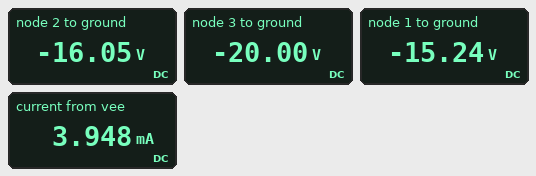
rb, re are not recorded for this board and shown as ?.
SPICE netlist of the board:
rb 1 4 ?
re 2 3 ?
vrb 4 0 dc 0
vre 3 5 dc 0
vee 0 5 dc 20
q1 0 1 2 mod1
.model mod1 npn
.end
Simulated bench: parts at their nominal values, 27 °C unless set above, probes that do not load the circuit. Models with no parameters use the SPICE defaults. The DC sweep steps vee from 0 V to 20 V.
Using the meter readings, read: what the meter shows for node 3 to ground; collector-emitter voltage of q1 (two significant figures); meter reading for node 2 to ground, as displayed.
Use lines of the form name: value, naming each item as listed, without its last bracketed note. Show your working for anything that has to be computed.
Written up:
what the meter shows for node 3 to ground: -20.00 V
collector-emitter voltage of q1: 0 V - (-16.05 V) = 16 V
meter reading for node 2 to ground, as displayed: -16.05 V
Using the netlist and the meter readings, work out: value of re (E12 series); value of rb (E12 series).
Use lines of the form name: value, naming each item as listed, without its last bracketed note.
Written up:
value of re: 1 kΩ
value of rb: 390 kΩ
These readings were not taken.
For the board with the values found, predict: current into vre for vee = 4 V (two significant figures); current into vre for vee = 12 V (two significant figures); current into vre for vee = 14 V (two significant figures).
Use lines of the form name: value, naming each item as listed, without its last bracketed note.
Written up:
current into vre for vee = 4 V: 670 µA
current into vre for vee = 12 V: 2.3 mA
current into vre for vee = 14 V: 2.7 mA
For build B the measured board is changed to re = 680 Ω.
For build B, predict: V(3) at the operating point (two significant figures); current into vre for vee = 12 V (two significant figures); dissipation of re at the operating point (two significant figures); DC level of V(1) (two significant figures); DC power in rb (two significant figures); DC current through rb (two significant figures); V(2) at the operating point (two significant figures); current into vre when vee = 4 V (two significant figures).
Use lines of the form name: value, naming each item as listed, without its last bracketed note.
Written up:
V(3) at the operating point: -20 V
current into vre for vee = 12 V: 2.5 mA
dissipation of re at the operating point: 12 mW
DC level of V(1): -16 V
DC power in rb: 680 µW
DC current through rb: 42 µA
V(2) at the operating point: -17 V
current into vre when vee = 4 V: 710 µA
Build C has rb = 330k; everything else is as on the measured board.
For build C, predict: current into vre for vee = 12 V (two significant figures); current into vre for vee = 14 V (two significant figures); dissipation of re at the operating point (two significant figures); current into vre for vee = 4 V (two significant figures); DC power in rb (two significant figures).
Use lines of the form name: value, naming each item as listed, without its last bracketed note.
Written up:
current into vre for vee = 12 V: 2.6 mA
current into vre for vee = 14 V: 3.1 mA
dissipation of re at the operating point: 20 mW
current into vre for vee = 4 V: 760 µA
DC power in rb: 650 µW
